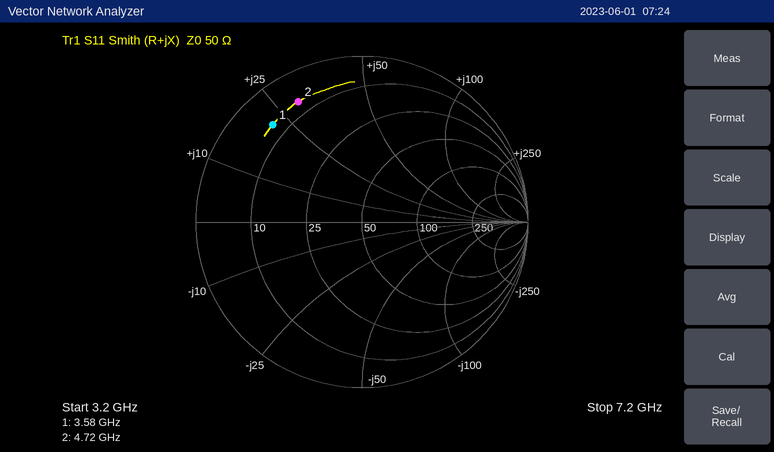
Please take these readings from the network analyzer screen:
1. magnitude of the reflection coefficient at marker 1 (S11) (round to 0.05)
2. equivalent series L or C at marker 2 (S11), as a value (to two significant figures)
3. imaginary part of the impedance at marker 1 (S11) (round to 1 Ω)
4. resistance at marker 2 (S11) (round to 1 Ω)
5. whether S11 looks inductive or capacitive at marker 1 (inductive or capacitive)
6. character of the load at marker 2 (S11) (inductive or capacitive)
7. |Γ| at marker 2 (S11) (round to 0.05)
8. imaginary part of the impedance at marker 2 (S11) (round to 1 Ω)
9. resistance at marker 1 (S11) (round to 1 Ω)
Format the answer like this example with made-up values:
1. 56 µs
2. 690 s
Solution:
1. 0.80
2. 1.0 nH
3. +22 Ω
4. 7 Ω
5. inductive
6. inductive
7. 0.80
8. +30 Ω
9. 7 Ω
